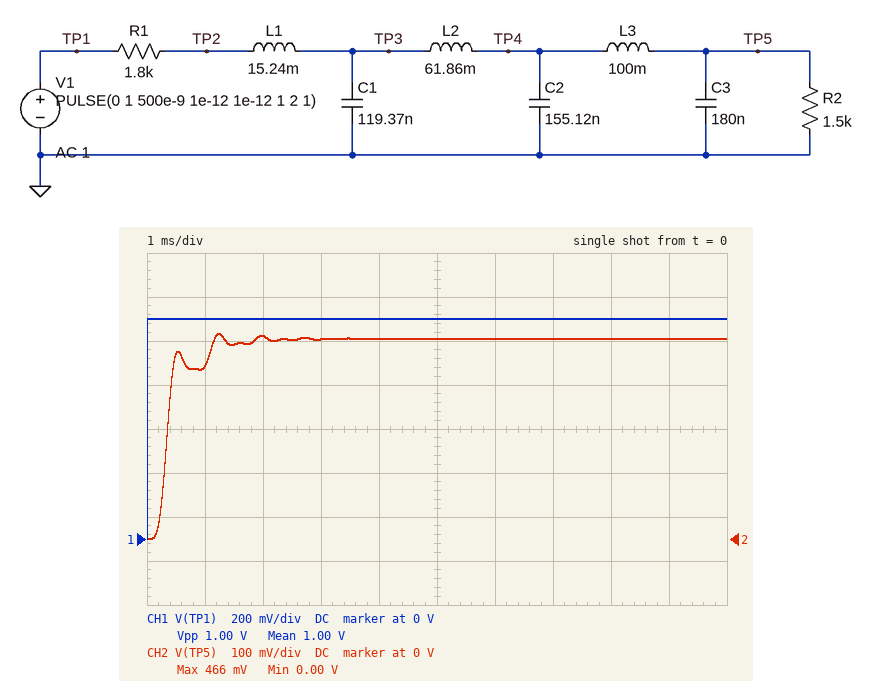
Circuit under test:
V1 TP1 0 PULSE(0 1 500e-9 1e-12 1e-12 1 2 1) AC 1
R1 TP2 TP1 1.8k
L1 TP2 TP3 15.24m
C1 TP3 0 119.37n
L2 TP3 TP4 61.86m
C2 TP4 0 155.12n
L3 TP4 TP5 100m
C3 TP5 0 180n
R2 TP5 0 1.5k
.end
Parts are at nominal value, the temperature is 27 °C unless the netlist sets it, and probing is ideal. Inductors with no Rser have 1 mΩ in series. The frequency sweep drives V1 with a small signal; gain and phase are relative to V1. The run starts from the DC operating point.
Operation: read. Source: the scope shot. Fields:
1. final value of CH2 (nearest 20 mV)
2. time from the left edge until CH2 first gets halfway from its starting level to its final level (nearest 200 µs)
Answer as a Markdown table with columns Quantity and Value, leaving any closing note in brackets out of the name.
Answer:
| Quantity | Value |
|---|---|
| final value of CH2 | 460 mV |
| time from the left edge until CH2 first gets halfway from its starting level to its final level | 400 µs |
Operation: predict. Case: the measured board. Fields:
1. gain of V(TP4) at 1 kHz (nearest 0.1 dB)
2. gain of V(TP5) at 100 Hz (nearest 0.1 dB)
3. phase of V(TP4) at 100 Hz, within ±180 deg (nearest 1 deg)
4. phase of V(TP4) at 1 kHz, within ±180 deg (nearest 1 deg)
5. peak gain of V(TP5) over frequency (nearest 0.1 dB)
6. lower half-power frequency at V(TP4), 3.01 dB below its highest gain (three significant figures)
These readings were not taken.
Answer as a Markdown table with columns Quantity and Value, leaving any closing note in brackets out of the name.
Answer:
| Quantity | Value |
|---|---|
| gain of V(TP4) at 1 kHz | -14.7 dB |
| gain of V(TP5) at 100 Hz | -7.0 dB |
| phase of V(TP4) at 100 Hz, within ±180 deg | -13 deg |
| phase of V(TP4) at 1 kHz, within ±180 deg | -47 deg |
| peak gain of V(TP5) over frequency | -6.8 dB |
| lower half-power frequency at V(TP4), 3.01 dB below its highest gain | 2.46 kHz |
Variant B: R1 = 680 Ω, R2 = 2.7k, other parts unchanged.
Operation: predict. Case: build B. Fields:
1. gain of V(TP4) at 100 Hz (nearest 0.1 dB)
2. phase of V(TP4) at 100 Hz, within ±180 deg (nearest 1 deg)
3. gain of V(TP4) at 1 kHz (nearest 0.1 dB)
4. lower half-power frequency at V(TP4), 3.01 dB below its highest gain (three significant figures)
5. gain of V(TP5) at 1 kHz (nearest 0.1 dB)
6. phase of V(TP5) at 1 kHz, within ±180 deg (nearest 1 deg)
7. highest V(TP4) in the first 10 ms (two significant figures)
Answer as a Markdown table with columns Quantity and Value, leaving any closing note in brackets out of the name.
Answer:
| Quantity | Value |
|---|---|
| gain of V(TP4) at 100 Hz | -2.0 dB |
| phase of V(TP4) at 100 Hz, within ±180 deg | -9 deg |
| gain of V(TP4) at 1 kHz | -10.1 dB |
| lower half-power frequency at V(TP4), 3.01 dB below its highest gain | 1.87 kHz |
| gain of V(TP5) at 1 kHz | -1.5 dB |
| phase of V(TP5) at 1 kHz, within ±180 deg | -111 deg |
| highest V(TP4) in the first 10 ms | 900 mV |
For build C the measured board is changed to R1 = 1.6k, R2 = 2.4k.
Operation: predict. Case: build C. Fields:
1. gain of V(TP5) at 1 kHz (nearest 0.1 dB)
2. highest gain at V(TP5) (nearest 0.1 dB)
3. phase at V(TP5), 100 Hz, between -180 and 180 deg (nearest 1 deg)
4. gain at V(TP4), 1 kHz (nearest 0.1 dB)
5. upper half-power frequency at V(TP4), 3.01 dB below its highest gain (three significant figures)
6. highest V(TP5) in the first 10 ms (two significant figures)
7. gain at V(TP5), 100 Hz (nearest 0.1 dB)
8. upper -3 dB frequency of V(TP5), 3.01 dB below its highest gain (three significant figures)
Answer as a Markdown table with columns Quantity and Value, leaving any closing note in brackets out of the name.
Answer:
| Quantity | Value |
|---|---|
| gain of V(TP5) at 1 kHz | -7.3 dB |
| highest gain at V(TP5) | -4.4 dB |
| phase at V(TP5), 100 Hz, between -180 and 180 deg | -17 deg |
| gain at V(TP4), 1 kHz | -15.5 dB |
| upper half-power frequency at V(TP4), 3.01 dB below its highest gain | 2.79 kHz |
| highest V(TP5) in the first 10 ms | 610 mV |
| gain at V(TP5), 100 Hz | -4.7 dB |
| upper -3 dB frequency of V(TP5), 3.01 dB below its highest gain | 1.62 kHz |
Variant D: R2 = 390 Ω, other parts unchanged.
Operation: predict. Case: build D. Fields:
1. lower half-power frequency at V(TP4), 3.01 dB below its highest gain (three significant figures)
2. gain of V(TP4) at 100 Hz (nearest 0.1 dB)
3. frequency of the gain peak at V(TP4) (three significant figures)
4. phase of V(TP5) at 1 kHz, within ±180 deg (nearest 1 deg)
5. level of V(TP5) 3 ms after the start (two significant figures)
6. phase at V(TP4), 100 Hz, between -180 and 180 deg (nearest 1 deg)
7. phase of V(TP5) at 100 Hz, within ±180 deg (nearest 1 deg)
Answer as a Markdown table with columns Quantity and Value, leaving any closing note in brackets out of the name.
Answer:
| Quantity | Value |
|---|---|
| lower half-power frequency at V(TP4), 3.01 dB below its highest gain | 2.41 kHz |
| gain of V(TP4) at 100 Hz | -14.9 dB |
| frequency of the gain peak at V(TP4) | 2.62 kHz |
| phase of V(TP5) at 1 kHz, within ±180 deg | -107 deg |
| level of V(TP5) 3 ms after the start | 180 mV |
| phase at V(TP4), 100 Hz, between -180 and 180 deg | 1 deg |
| phase of V(TP5) at 100 Hz, within ±180 deg | -8 deg |
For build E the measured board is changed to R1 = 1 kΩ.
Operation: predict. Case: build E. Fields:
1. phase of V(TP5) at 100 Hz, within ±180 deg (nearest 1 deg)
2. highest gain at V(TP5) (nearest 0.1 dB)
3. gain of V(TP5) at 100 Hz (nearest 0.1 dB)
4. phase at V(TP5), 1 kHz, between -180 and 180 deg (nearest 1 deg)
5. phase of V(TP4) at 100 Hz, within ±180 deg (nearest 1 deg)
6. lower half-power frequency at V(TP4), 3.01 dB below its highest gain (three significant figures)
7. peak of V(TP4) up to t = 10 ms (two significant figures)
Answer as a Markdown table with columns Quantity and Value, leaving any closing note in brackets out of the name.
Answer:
| Quantity | Value |
|---|---|
| phase of V(TP5) at 100 Hz, within ±180 deg | -12 deg |
| highest gain at V(TP5) | -4.4 dB |
| gain of V(TP5) at 100 Hz | -4.5 dB |
| phase at V(TP5), 1 kHz, between -180 and 180 deg | -106 deg |
| phase of V(TP4) at 100 Hz, within ±180 deg | -10 deg |
| lower half-power frequency at V(TP4), 3.01 dB below its highest gain | 2.18 kHz |
| peak of V(TP4) up to t = 10 ms | 630 mV |
